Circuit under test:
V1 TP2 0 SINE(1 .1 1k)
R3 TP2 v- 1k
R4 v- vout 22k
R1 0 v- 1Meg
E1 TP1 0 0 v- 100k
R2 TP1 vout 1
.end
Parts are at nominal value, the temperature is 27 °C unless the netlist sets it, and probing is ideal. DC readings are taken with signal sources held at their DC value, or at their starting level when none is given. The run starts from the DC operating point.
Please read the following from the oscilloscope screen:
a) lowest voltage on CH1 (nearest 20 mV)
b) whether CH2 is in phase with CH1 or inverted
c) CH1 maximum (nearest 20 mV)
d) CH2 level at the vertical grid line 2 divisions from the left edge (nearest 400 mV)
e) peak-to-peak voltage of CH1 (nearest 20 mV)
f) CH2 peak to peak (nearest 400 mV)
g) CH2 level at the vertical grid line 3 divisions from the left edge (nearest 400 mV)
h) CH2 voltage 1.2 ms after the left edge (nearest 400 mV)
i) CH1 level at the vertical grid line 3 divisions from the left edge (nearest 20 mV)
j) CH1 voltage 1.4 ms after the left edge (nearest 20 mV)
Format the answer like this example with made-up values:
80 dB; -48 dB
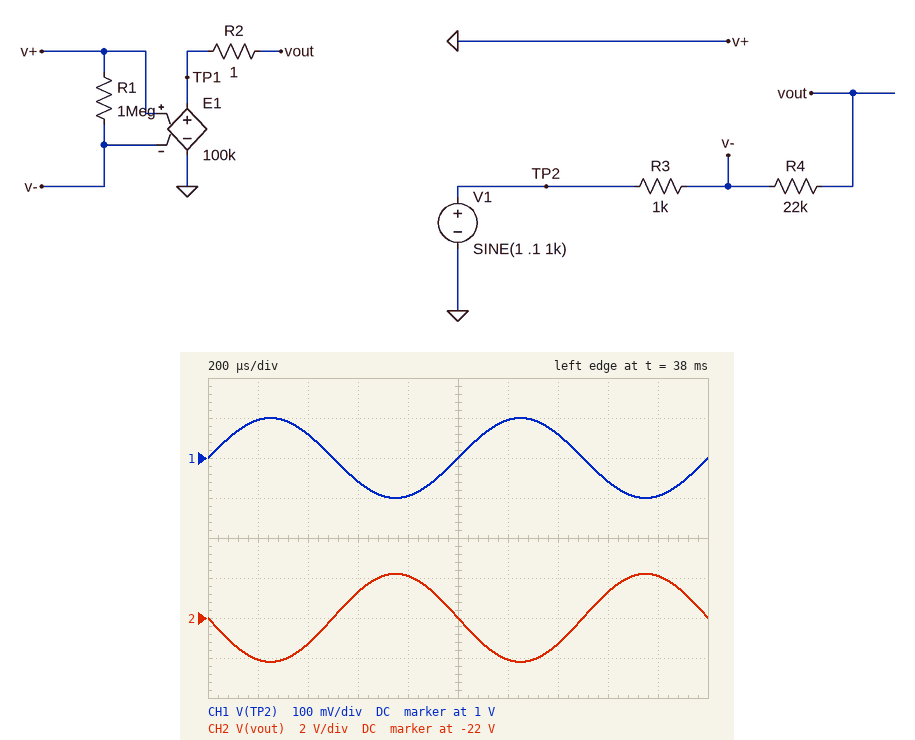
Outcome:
900 mV; inverted; 1.10 V; -23.2 V; 200 mV; 4.4 V; -20.8 V; -24.0 V; 940 mV; 1.06 V
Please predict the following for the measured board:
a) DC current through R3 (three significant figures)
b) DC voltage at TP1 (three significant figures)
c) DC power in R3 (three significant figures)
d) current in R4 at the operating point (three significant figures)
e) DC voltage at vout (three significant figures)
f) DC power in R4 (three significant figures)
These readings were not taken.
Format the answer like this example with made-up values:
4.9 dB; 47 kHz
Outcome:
1.00 mA; -22.0 V; 1.00 mW; 1.00 mA; -22.0 V; 22.0 mW
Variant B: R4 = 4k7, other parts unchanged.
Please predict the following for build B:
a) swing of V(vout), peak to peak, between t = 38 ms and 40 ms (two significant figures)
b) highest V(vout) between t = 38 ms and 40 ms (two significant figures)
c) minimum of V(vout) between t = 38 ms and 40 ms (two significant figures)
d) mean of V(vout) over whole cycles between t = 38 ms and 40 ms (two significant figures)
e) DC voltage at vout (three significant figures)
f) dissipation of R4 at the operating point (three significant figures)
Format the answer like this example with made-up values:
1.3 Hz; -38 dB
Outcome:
940 mV; -4.2 V; -5.2 V; -4.7 V; -4.70 V; 4.70 mW
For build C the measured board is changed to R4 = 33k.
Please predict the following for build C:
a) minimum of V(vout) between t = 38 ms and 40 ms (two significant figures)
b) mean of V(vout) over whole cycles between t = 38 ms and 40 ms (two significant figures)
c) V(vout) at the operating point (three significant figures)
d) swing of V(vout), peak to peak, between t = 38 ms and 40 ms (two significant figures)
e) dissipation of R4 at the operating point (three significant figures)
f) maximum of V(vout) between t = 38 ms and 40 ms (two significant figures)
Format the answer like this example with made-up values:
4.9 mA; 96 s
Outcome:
-36 V; -33 V; -33.0 V; 6.6 V; 33.0 mW; -30 V
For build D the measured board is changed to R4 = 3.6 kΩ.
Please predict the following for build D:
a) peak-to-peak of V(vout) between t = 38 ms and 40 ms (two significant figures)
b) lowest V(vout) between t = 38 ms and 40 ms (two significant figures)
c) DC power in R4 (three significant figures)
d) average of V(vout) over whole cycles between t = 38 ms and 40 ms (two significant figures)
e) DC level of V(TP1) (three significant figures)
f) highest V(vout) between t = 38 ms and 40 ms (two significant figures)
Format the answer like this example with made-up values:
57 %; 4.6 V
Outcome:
720 mV; -4.0 V; 3.60 mW; -3.6 V; -3.60 V; -3.2 V
